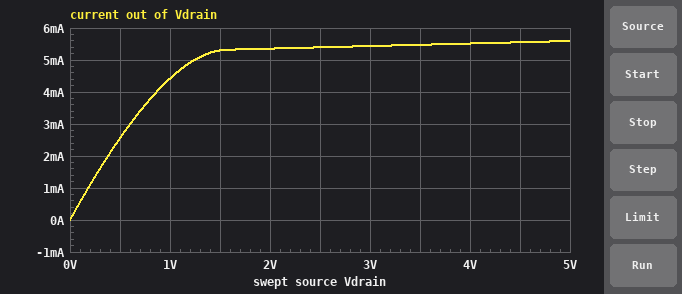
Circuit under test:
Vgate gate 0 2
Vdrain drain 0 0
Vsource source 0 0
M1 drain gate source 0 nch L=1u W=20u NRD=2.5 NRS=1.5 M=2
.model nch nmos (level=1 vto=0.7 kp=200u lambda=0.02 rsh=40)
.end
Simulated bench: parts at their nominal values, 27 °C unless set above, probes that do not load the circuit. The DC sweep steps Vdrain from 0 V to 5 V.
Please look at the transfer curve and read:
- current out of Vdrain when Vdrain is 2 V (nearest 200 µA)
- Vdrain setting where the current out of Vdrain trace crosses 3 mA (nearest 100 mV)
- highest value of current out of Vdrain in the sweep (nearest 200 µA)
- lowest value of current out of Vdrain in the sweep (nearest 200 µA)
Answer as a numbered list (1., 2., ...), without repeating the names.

1. 5.4 mA
2. 600 mV
3. 5.6 mA
4. 0 A
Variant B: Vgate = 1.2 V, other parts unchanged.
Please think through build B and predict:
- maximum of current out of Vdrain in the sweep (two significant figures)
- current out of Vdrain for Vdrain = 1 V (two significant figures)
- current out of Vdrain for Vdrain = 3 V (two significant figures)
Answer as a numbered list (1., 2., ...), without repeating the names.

1. 970 µA
2. 910 µA
3. 940 µA
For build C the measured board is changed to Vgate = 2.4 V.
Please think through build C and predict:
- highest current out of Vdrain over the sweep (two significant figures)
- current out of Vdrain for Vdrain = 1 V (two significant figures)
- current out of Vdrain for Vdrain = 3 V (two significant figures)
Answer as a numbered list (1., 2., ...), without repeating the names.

1. 8.9 mA
2. 5.6 mA
3. 8.7 mA
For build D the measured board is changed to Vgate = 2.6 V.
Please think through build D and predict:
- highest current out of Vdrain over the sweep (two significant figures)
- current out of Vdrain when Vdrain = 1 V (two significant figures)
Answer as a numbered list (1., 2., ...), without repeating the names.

1. 11 mA
2. 6.1 mA
